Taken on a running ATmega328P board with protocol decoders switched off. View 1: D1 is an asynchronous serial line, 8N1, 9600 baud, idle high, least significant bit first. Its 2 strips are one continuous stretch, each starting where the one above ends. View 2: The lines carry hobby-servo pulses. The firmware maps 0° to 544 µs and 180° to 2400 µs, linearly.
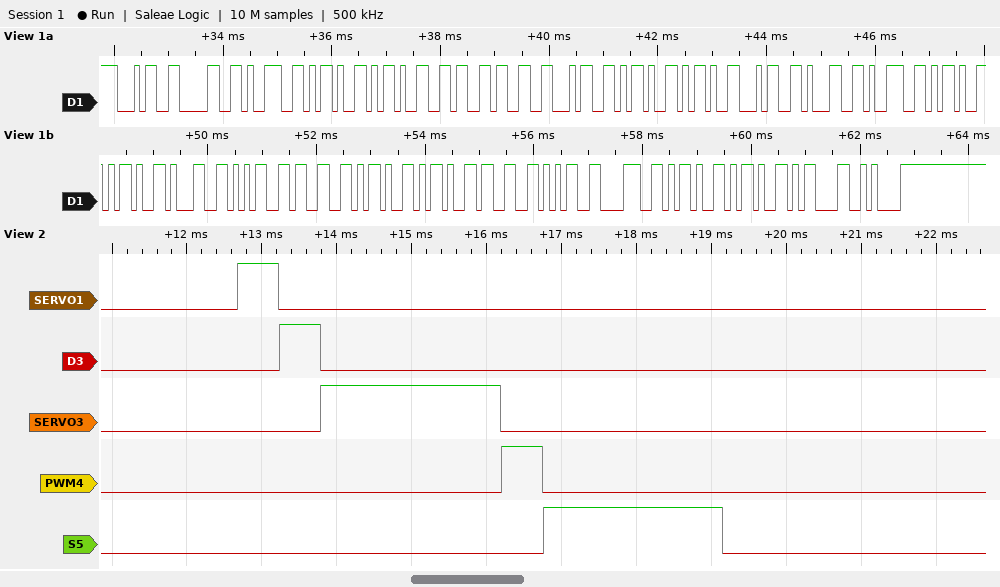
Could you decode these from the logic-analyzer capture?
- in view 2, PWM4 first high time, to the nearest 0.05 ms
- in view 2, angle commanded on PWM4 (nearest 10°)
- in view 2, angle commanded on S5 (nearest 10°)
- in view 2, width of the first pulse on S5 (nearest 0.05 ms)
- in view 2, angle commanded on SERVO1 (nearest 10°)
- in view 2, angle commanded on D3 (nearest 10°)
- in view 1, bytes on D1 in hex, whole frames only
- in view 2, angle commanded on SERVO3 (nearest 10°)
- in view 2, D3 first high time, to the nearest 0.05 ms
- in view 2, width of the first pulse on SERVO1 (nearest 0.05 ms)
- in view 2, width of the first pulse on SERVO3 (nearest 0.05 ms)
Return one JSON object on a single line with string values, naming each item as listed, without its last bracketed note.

{"in view 2, PWM4 first high time, to the nearest 0.05 ms": "0.55 ms", "in view 2, angle commanded on PWM4": "0°", "in view 2, angle commanded on S5": "180°", "in view 2, width of the first pulse on S5": "2.40 ms", "in view 2, angle commanded on SERVO1": "0°", "in view 2, angle commanded on D3": "0°", "in view 1, bytes on D1 in hex, whole frames only": "0x34 0x30 0x39 0x2D 0x2D 0x36 0x33 0x34 0x2D 0x2D 0x34 0x31 0x39 0x2D 0x2D 0x31 0x35 0x33 0x2D 0x2D 0x33 0x35 0x38 0x2D 0x2D 0x0D 0x0A", "in view 2, angle commanded on SERVO3": "180°", "in view 2, D3 first high time, to the nearest 0.05 ms": "0.55 ms", "in view 2, width of the first pulse on SERVO1": "0.55 ms", "in view 2, width of the first pulse on SERVO3": "2.40 ms"}
